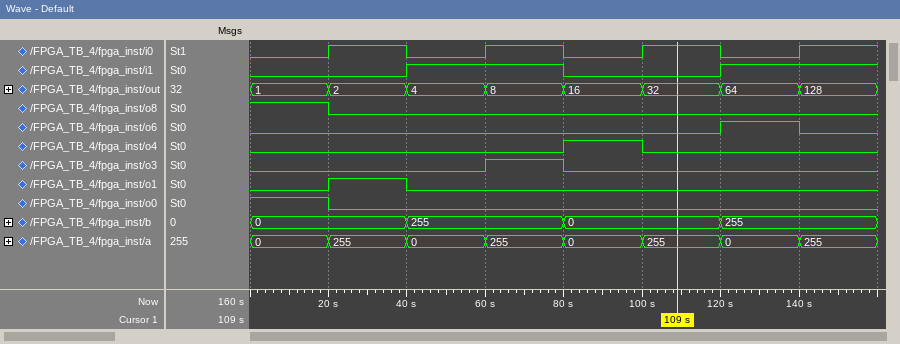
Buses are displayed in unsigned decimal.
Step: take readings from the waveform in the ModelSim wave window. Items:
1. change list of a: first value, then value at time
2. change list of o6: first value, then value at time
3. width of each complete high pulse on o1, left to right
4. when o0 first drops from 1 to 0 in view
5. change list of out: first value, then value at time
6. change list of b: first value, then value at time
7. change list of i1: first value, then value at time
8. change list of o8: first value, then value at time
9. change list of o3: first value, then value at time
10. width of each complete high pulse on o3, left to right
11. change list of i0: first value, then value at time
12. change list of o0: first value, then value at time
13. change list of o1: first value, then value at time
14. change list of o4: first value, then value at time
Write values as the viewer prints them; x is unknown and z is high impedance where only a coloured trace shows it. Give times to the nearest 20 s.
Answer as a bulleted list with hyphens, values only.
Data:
- 0, 255 at 20 s, 0 at 40 s, 255 at 60 s, 0 at 80 s, 255 at 100 s, 0 at 120 s, 255 at 140 s
- 0, 1 at 120 s, 0 at 140 s
- 20 s
- 20 s
- 1, 2 at 20 s, 4 at 40 s, 8 at 60 s, 16 at 80 s, 32 at 100 s, 64 at 120 s, 128 at 140 s
- 0, 255 at 40 s, 0 at 80 s, 255 at 120 s
- 0, 1 at 40 s, 0 at 80 s, 1 at 120 s
- 1, 0 at 20 s
- 0, 1 at 60 s, 0 at 80 s
- 20 s
- 0, 1 at 20 s, 0 at 40 s, 1 at 60 s, 0 at 80 s, 1 at 100 s, 0 at 120 s, 1 at 140 s
- 1, 0 at 20 s
- 0, 1 at 20 s, 0 at 40 s
- 0, 1 at 80 s, 0 at 100 s
